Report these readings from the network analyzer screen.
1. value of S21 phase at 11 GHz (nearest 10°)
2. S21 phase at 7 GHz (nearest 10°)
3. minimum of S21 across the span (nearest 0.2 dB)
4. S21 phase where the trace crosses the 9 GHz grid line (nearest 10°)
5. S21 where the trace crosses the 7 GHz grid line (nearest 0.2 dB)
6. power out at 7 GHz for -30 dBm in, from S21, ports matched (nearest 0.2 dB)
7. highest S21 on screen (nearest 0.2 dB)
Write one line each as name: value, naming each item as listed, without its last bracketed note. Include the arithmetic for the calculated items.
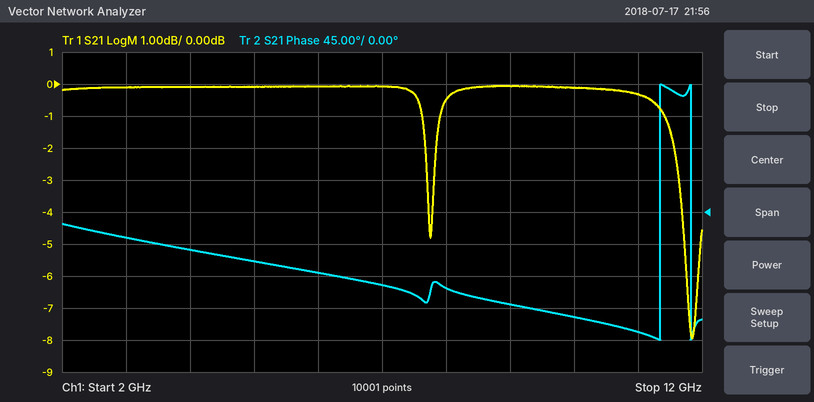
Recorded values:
value of S21 phase at 11 GHz: -170°
S21 phase at 7 GHz: -100°
minimum of S21 across the span: -8.0 dB
S21 phase where the trace crosses the 9 GHz grid line: -130°
S21 where the trace crosses the 7 GHz grid line: 0.0 dB
power out at 7 GHz for -30 dBm in, from S21, ports matched: -30 dBm + (0.0 dB) = -30.0 dBm
highest S21 on screen: 0.0 dB
